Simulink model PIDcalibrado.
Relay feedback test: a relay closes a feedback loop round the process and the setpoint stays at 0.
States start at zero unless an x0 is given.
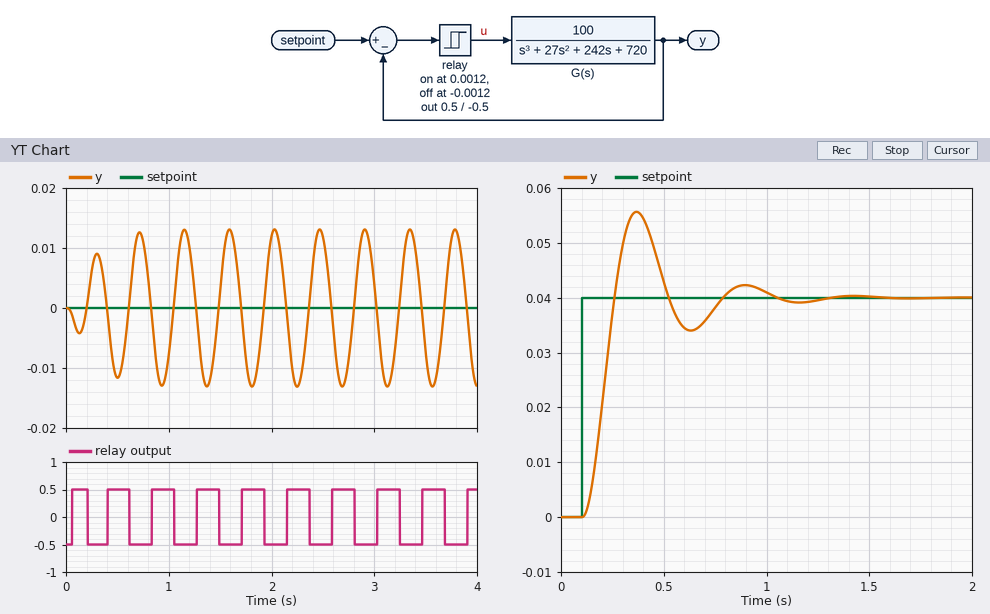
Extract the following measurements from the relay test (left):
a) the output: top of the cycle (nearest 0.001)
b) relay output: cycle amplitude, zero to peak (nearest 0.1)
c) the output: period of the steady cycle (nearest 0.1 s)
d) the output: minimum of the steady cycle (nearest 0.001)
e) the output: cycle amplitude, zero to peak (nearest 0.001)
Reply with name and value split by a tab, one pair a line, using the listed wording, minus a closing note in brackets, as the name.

the output: top of the cycle	0.013
relay output: cycle amplitude, zero to peak	0.5
the output: period of the steady cycle	0.4 s
the output: minimum of the steady cycle	-0.013
the output: cycle amplitude, zero to peak	0.013
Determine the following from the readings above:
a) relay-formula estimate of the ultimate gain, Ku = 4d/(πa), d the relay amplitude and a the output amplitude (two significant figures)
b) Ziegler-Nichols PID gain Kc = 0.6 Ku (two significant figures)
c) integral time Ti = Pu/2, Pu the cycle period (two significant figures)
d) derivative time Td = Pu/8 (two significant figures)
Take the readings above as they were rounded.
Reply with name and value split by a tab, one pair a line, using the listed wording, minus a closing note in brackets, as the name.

relay-formula estimate of the ultimate gain, Ku = 4d/(πa), d the relay amplitude and a the output amplitude	49
Ziegler-Nichols PID gain Kc = 0.6 Ku	29
integral time Ti = Pu/2, Pu the cycle period	0.20 s
derivative time Td = Pu/8	0.050 s
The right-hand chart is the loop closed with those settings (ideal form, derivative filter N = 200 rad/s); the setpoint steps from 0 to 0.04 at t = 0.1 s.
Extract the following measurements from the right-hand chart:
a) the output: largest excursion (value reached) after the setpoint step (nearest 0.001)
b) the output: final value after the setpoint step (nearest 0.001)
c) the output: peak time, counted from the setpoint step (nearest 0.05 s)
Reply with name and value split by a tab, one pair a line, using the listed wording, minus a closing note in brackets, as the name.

the output: largest excursion (value reached) after the setpoint step	0.056
the output: final value after the setpoint step	0.040
the output: peak time, counted from the setpoint step	0.25 s
